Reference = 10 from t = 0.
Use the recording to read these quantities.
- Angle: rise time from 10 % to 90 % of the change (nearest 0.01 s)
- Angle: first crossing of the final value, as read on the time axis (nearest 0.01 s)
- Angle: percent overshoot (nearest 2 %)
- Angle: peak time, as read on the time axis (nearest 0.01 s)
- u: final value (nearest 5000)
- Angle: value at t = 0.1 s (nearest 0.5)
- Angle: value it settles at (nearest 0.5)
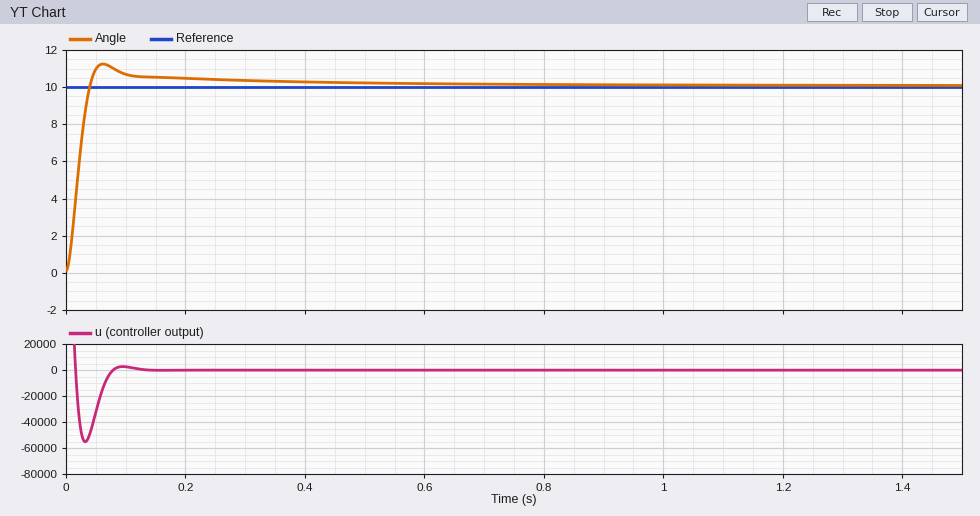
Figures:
0.03 s
0.04 s
12 %
0.06 s
0
10.5
10.0
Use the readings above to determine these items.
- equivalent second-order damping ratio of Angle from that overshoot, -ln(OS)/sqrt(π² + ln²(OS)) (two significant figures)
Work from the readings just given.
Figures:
0.56
